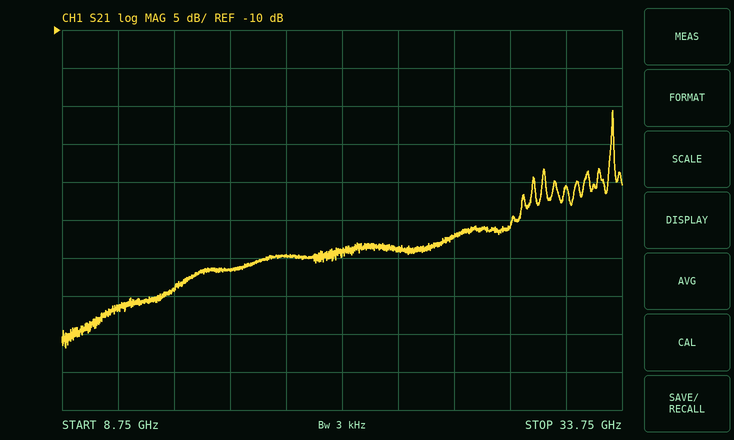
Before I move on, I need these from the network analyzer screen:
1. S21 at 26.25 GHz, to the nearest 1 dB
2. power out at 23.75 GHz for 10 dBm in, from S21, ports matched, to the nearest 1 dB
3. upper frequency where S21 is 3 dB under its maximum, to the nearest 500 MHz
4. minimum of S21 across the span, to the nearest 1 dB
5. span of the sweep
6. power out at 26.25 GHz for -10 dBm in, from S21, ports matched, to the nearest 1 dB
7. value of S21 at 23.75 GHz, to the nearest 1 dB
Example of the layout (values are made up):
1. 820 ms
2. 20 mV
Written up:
1. -37 dB
2. -29 dBm
3. 33.5 GHz
4. -52 dB
5. 25 GHz
6. -47 dBm
7. -39 dB
